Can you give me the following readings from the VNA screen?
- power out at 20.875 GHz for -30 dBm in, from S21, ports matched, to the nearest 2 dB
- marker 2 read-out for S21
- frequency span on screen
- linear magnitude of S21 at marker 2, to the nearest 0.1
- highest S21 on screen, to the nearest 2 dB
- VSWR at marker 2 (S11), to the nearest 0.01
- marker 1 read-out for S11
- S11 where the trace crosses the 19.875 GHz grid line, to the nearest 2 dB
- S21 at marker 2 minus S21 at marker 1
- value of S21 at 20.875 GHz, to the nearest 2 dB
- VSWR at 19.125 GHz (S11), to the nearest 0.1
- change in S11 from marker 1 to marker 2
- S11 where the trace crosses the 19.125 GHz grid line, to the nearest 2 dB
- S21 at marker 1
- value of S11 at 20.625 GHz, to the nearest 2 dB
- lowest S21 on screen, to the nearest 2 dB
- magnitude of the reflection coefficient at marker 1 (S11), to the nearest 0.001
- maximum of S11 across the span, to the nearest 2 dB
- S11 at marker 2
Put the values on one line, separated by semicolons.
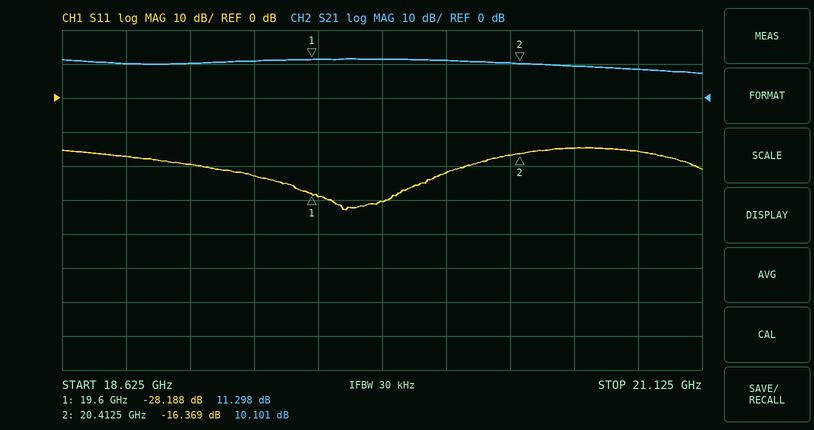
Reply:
-22 dBm; 10.101 dB; 2.5 GHz; 3.2; 12 dB; 1.36; -28.188 dB; -30 dB; -1.197 dB; 8 dB; 1.2; 11.819 dB; -20 dB; 11.298 dB; -14 dB; 8 dB; 0.039; -14 dB; -16.369 dB
